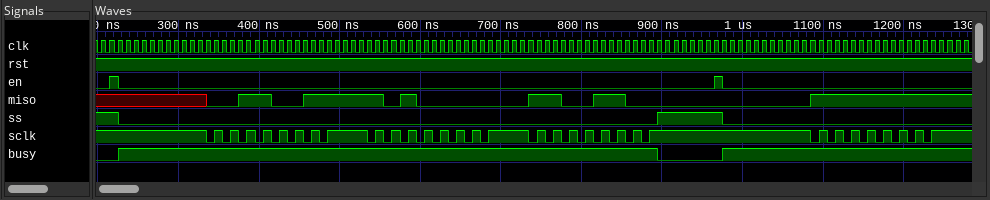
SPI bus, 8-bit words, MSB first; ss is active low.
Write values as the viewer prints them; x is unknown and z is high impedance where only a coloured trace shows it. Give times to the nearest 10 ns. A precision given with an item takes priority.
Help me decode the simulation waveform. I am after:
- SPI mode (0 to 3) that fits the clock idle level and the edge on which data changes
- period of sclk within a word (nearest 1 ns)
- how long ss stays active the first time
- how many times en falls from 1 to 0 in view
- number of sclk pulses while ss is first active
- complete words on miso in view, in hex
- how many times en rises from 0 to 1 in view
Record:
3
20 ns
670 ns
2
24
33, A0, CC, FF
2
